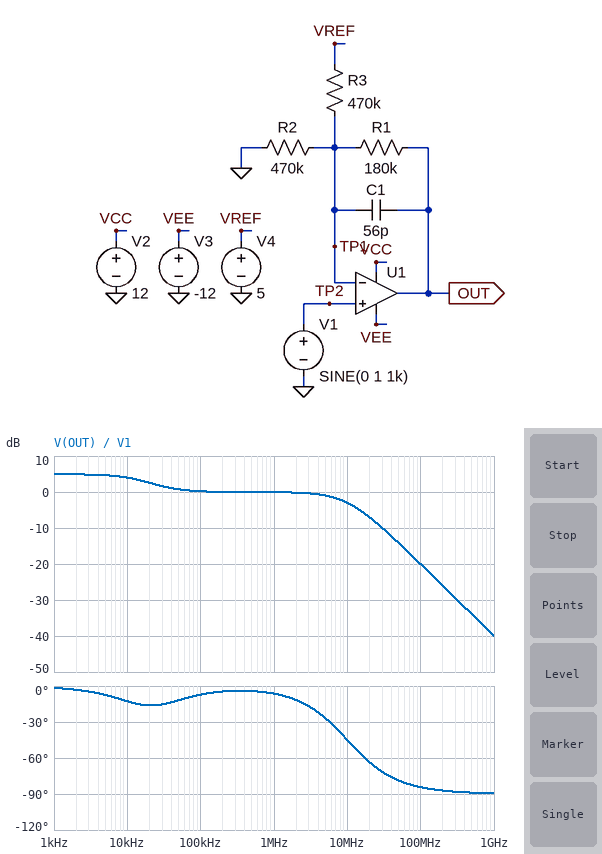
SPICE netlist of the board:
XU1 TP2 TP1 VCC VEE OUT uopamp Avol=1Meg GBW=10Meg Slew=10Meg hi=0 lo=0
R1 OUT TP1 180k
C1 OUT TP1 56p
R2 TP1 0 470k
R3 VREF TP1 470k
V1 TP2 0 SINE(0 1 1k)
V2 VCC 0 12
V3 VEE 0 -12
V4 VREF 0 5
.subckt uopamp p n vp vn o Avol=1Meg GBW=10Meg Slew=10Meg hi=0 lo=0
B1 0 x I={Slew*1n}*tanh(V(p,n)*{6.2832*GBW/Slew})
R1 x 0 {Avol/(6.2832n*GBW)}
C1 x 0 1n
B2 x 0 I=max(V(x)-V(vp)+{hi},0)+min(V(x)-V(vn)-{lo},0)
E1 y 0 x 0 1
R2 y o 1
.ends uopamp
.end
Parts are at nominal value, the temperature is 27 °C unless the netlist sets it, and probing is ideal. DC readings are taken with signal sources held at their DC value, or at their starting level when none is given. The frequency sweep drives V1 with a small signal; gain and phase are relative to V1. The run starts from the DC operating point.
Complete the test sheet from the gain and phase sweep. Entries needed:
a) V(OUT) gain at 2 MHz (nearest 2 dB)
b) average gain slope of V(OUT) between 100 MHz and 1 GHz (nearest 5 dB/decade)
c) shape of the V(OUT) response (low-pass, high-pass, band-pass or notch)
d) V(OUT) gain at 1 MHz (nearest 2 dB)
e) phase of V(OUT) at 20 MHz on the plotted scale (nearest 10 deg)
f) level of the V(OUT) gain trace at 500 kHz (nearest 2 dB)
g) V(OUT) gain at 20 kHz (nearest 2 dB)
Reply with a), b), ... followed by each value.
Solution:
a) 0 dB
b) -20 dB/decade
c) low-pass
d) 0 dB
e) -60 deg
f) 0 dB
g) 2 dB
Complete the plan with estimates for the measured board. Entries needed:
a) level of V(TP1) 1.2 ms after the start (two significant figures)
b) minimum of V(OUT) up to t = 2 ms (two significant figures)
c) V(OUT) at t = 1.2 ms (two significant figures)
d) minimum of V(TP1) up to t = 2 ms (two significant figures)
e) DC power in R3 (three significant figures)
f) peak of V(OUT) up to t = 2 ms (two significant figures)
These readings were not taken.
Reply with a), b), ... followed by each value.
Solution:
a) 950 mV
b) -3.7 V
c) -250 mV
d) -1.0 V
e) 53.2 µW
f) -150 mV
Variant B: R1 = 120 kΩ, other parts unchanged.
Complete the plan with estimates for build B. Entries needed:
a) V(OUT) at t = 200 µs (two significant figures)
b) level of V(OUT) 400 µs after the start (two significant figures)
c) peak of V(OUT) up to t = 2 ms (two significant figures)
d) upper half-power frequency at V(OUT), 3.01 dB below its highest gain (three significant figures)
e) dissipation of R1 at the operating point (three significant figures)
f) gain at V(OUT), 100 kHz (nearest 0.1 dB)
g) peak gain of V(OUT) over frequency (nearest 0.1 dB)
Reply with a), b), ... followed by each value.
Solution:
a) 150 mV
b) -370 mV
c) 230 mV
d) 66.7 kHz
e) 13.6 µW
f) 0.3 dB
g) 3.6 dB
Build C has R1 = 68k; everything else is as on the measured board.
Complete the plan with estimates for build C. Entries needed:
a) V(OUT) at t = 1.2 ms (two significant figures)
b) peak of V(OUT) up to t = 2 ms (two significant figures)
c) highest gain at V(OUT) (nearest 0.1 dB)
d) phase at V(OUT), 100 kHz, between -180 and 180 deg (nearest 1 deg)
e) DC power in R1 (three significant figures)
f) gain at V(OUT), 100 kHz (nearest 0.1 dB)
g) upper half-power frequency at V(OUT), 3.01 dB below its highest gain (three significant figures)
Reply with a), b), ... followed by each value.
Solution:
a) 500 mV
b) 570 mV
c) 2.2 dB
d) -6 deg
e) 7.70 µW
f) 0.4 dB
g) 4.48 MHz
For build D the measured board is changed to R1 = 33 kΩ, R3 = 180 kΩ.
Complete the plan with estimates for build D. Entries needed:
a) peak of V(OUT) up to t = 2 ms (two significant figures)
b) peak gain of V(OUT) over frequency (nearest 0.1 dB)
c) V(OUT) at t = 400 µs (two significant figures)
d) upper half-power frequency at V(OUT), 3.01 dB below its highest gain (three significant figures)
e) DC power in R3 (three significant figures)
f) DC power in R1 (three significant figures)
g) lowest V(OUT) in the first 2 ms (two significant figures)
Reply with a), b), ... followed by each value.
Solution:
a) 340 mV
b) 2.0 dB
c) -180 mV
d) 5.18 MHz
e) 139 µW
f) 25.5 µW
g) -2.2 V
